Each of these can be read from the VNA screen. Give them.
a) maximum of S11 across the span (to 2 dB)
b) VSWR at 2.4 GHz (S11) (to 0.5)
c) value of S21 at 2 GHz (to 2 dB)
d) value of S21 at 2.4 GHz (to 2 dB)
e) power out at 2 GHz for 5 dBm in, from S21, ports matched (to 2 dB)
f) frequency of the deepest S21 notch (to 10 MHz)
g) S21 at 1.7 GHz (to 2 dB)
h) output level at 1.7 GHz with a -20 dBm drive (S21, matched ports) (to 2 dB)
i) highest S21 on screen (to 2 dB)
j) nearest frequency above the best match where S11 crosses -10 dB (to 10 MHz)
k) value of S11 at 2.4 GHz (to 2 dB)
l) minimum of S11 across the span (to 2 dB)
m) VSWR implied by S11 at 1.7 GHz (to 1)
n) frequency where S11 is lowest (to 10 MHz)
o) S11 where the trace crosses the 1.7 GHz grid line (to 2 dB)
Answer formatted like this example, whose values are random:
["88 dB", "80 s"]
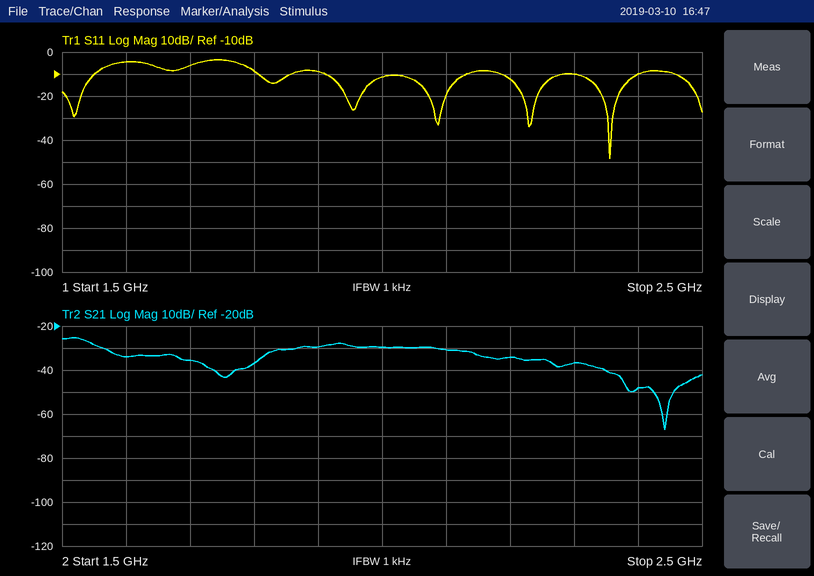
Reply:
["-4 dB", "2.0", "-30 dB", "-48 dB", "-24 dBm", "2.44 GHz", "-36 dB", "-56 dBm", "-26 dB", "2.40 GHz", "-10 dB", "-48 dB", "3", "2.36 GHz", "-6 dB"]
